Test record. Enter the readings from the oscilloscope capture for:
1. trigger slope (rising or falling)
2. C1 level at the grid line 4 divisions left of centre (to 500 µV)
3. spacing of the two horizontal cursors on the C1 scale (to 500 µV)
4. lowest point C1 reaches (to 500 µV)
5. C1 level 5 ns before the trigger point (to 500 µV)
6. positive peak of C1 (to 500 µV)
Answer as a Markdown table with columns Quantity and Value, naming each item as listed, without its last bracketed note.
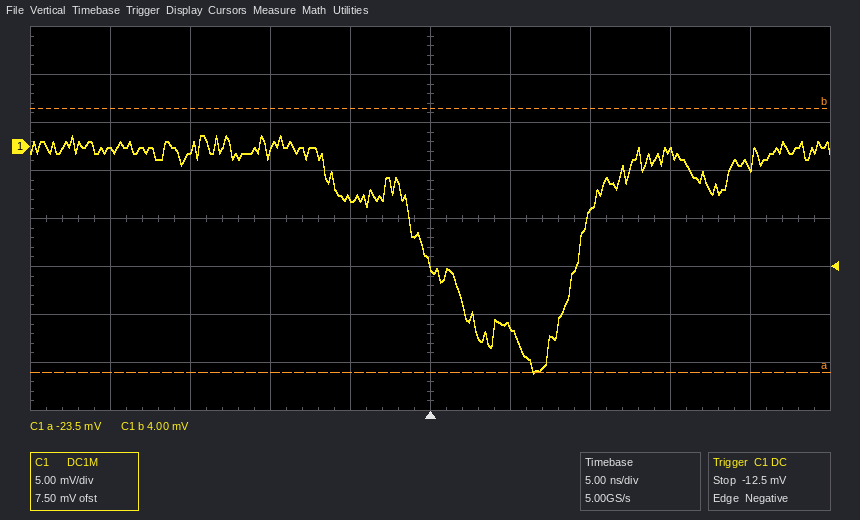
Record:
| Quantity | Value |
|---|---|
| trigger slope | falling |
| C1 level at the grid line 4 divisions left of centre | -500 µV |
| spacing of the two horizontal cursors on the C1 scale | 27.5 mV |
| lowest point C1 reaches | -23.5 mV |
| C1 level 5 ns before the trigger point | -5.5 mV |
| positive peak of C1 | 1.0 mV |
